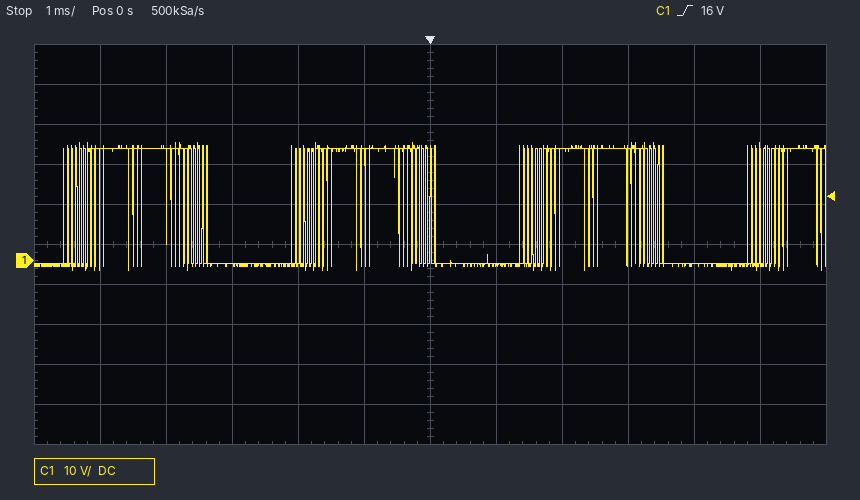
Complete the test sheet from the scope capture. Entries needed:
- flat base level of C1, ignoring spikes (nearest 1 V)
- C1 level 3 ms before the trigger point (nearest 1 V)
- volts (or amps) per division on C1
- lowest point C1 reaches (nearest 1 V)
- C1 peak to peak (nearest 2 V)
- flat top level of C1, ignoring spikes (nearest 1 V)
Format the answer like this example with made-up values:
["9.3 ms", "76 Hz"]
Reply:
["-1 V", "-1 V", "10 V", "-2 V", "32 V", "28 V"]
